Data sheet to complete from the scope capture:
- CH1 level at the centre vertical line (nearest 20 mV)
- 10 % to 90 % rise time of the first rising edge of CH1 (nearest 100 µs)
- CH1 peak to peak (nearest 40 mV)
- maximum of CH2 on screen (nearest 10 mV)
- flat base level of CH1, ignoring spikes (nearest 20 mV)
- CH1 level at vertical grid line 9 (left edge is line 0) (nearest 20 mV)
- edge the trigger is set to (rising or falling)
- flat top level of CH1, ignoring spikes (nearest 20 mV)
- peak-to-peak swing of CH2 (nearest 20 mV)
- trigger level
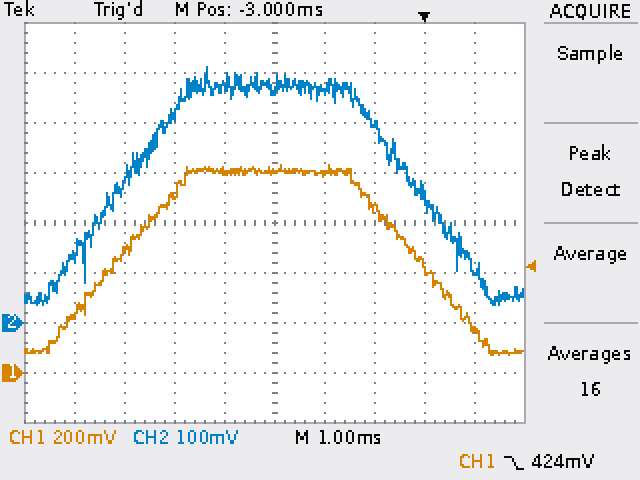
800 mV
2.4 ms
760 mV
510 mV
80 mV
180 mV
falling
800 mV
480 mV
424 mV
